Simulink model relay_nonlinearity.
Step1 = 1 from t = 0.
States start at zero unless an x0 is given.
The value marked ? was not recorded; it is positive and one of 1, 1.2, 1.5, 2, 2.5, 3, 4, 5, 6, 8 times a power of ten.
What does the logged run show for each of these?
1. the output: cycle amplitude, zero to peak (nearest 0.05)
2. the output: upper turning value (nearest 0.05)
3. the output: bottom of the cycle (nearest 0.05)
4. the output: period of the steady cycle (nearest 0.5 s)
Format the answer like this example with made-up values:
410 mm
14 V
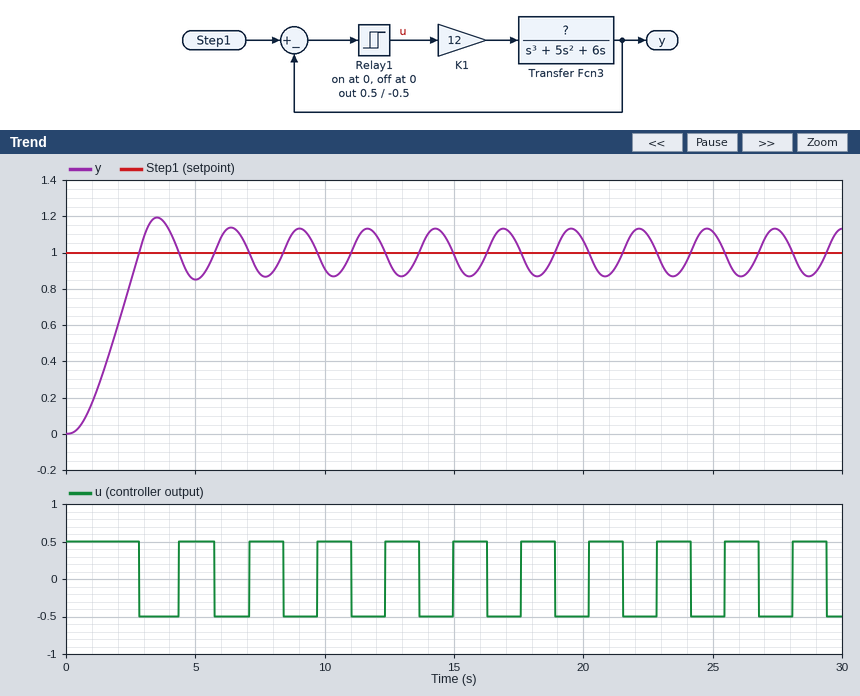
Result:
0.15
1.15
0.85
2.5 s
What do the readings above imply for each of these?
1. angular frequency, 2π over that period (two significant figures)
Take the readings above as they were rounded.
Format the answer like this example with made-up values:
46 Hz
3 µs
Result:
2.5 rad/s
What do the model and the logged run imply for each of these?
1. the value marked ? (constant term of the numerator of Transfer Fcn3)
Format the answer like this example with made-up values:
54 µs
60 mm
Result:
0.5
